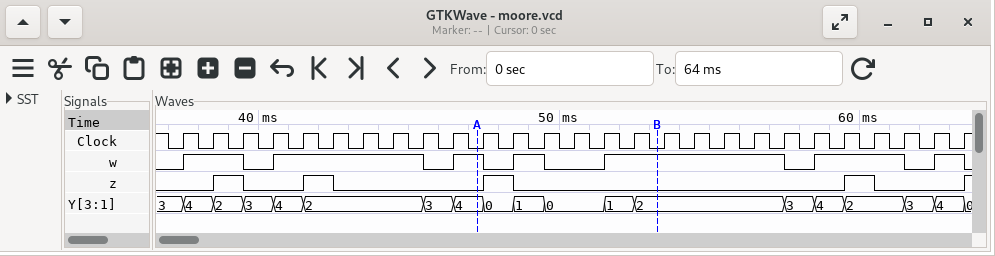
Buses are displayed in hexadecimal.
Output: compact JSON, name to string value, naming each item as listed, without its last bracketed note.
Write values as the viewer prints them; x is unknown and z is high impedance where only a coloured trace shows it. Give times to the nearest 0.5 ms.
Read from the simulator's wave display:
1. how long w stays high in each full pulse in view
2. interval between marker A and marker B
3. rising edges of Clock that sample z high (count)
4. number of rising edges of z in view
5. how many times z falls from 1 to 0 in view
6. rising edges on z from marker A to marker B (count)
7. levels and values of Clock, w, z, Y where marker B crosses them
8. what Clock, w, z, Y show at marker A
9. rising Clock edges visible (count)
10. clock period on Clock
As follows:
{"how long w stays high in each full pulse in view": "2 ms, 5 ms, 1 ms, 1 ms, 6 ms, 3 ms, 1 ms", "interval between marker A and marker B": "6 ms", "rising edges of Clock that sample z high": "4", "number of rising edges of z in view": "5", "how many times z falls from 1 to 0 in view": "4", "rising edges on z from marker A to marker B": "1", "levels and values of Clock, w, z, Y where marker B crosses them": "Clock=0, w=1, z=0, Y=2", "what Clock, w, z, Y show at marker A": "Clock=0, w=1, z=0, Y=4", "rising Clock edges visible": "27", "clock period on Clock": "1 ms"}
